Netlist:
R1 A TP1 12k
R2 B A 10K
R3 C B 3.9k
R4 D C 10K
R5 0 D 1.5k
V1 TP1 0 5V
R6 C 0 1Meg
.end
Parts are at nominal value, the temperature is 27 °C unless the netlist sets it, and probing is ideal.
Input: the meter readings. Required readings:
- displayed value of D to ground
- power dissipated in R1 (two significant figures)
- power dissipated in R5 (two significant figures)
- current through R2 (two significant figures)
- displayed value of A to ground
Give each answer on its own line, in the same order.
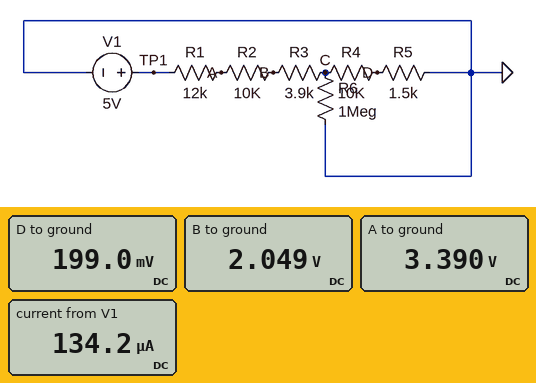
199.0 mV
220 µW
26 µW
130 µA
3.390 V
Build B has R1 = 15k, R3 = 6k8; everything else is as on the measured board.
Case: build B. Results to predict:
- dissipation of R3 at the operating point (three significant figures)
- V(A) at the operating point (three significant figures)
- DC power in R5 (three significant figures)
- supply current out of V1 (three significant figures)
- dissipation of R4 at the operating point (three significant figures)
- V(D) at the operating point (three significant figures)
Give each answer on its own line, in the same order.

91.2 µW
3.26 V
19.7 µW
116 µA
131 µW
172 mV
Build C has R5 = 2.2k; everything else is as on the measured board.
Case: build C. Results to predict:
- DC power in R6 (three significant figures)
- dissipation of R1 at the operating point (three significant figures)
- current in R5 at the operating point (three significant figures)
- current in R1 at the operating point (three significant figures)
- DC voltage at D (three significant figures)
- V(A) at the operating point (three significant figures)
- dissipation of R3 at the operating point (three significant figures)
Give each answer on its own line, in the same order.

2.52 µW
208 µW
130 µA
132 µA
286 mV
3.42 V
67.7 µW
